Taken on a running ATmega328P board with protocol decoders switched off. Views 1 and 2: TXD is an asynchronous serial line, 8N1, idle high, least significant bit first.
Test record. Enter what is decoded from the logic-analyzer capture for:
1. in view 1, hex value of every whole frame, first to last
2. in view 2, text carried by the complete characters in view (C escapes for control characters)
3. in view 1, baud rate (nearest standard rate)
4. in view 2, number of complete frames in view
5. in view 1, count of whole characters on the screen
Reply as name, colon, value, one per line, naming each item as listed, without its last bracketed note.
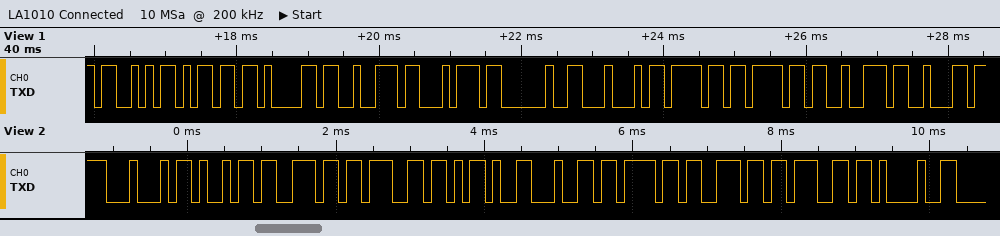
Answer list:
in view 1, hex value of every whole frame, first to last: 0x53 0x6D 0x61 0x72 0x74 0x20 0x44 0x6F 0x6F 0x72 0x62
in view 2, text carried by the complete characters in view: "Ding-dong!"
in view 1, baud rate: 9600 baud
in view 2, number of complete frames in view: 10
in view 1, count of whole characters on the screen: 11
